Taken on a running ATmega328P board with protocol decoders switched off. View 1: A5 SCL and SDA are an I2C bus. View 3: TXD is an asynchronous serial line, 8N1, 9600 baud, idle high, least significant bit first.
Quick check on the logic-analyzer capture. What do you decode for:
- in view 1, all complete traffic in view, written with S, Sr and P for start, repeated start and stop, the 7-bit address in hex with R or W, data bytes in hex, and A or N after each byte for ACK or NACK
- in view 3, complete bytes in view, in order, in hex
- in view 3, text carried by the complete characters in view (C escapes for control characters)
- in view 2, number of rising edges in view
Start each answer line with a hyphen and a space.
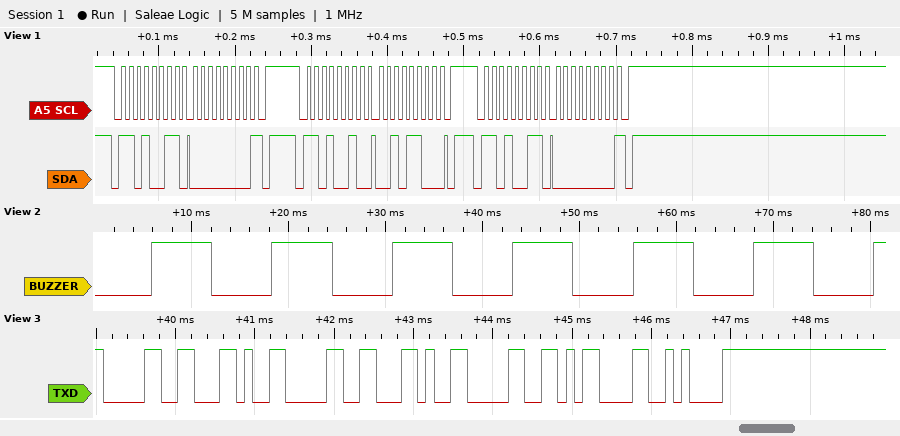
- S 69R A 00 N P S 69W A 2C A P S 69R A 00 N P
- 30 2C 30 2C 30 0D 0A
- "0,0,0\r\n"
- 7
